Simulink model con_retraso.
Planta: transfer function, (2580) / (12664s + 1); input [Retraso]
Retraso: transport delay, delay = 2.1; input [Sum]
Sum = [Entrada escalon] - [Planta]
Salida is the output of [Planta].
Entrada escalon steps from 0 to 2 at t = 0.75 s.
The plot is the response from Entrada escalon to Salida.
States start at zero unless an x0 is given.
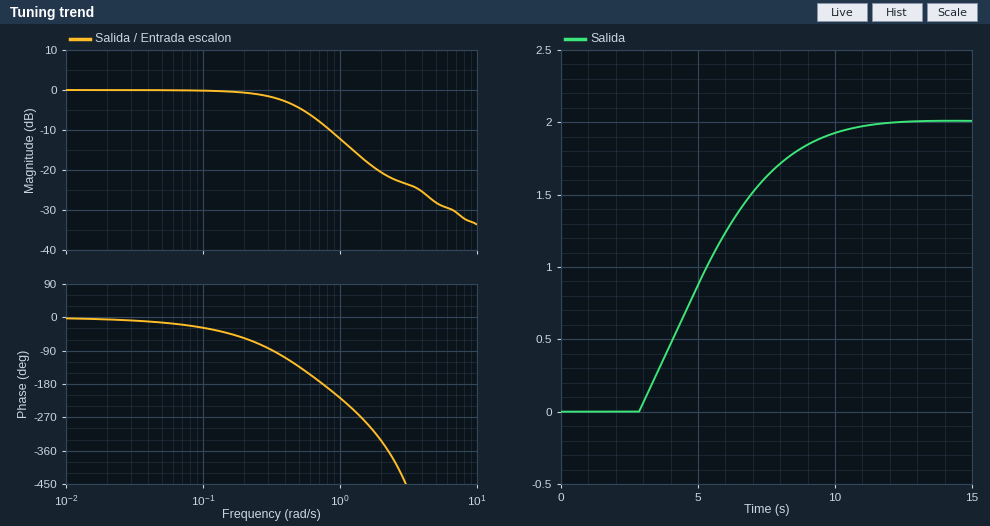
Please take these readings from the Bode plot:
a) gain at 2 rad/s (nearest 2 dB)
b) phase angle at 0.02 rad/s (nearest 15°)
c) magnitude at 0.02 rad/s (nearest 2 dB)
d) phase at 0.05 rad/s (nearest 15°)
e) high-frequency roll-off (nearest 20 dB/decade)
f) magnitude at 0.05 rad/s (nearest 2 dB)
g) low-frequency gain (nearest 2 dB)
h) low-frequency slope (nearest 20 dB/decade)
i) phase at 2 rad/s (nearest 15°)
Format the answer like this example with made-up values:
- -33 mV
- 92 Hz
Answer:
- -20 dB
- 0°
- 0 dB
- -15°
- -20 dB/decade
- 0 dB
- 0 dB
- 0 dB/decade
- -330°
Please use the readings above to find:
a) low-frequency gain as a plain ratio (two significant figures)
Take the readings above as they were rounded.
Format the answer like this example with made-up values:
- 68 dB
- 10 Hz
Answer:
- 1.0
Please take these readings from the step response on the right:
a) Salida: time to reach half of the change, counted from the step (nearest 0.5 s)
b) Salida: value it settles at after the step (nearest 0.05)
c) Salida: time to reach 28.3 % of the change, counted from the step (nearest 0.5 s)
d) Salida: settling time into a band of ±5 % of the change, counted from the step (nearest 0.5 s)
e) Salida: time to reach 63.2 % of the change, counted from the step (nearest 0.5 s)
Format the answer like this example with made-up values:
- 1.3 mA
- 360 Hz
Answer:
- 4.5 s
- 2.00
- 3.5 s
- 9.0 s
- 5.5 s
